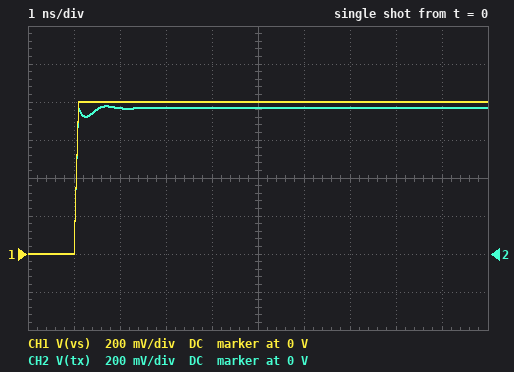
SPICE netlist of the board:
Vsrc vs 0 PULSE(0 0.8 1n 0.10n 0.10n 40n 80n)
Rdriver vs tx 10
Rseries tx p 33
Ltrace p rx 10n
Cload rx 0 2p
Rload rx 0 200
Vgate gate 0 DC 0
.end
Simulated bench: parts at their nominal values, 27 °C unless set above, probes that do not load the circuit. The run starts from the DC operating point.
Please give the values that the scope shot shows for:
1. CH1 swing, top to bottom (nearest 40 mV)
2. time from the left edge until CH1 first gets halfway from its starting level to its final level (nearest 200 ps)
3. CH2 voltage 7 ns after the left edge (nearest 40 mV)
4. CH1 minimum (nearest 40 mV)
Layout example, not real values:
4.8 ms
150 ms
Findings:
800 mV
1.0 ns
760 mV
0 V
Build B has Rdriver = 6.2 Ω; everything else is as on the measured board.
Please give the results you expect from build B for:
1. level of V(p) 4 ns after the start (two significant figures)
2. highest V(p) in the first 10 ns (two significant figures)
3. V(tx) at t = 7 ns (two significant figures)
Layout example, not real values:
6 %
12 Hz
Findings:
670 mV
710 mV
780 mV
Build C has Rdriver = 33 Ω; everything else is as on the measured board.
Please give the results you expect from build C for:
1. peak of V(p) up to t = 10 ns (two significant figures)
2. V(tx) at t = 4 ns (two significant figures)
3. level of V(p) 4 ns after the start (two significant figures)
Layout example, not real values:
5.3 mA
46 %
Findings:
630 mV
700 mV
600 mV
